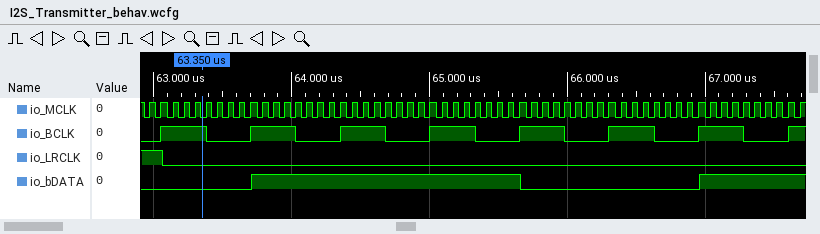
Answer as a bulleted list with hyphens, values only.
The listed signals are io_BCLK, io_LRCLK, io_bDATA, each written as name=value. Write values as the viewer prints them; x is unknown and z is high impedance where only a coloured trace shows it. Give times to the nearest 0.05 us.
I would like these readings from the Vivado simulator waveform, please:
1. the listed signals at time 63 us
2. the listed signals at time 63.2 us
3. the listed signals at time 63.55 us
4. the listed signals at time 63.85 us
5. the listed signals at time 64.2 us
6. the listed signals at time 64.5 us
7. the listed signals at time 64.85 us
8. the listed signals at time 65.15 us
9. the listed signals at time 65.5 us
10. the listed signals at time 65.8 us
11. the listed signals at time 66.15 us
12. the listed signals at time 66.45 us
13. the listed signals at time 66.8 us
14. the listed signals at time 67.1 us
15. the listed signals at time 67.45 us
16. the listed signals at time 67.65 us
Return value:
- io_BCLK=0, io_LRCLK=1, io_bDATA=0
- io_BCLK=1, io_LRCLK=0, io_bDATA=0
- io_BCLK=0, io_LRCLK=0, io_bDATA=0
- io_BCLK=1, io_LRCLK=0, io_bDATA=1
- io_BCLK=0, io_LRCLK=0, io_bDATA=1
- io_BCLK=1, io_LRCLK=0, io_bDATA=1
- io_BCLK=0, io_LRCLK=0, io_bDATA=1
- io_BCLK=1, io_LRCLK=0, io_bDATA=1
- io_BCLK=0, io_LRCLK=0, io_bDATA=1
- io_BCLK=1, io_LRCLK=0, io_bDATA=0
- io_BCLK=0, io_LRCLK=0, io_bDATA=0
- io_BCLK=1, io_LRCLK=0, io_bDATA=0
- io_BCLK=0, io_LRCLK=0, io_bDATA=0
- io_BCLK=1, io_LRCLK=0, io_bDATA=1
- io_BCLK=0, io_LRCLK=0, io_bDATA=1
- io_BCLK=1, io_LRCLK=0, io_bDATA=1
